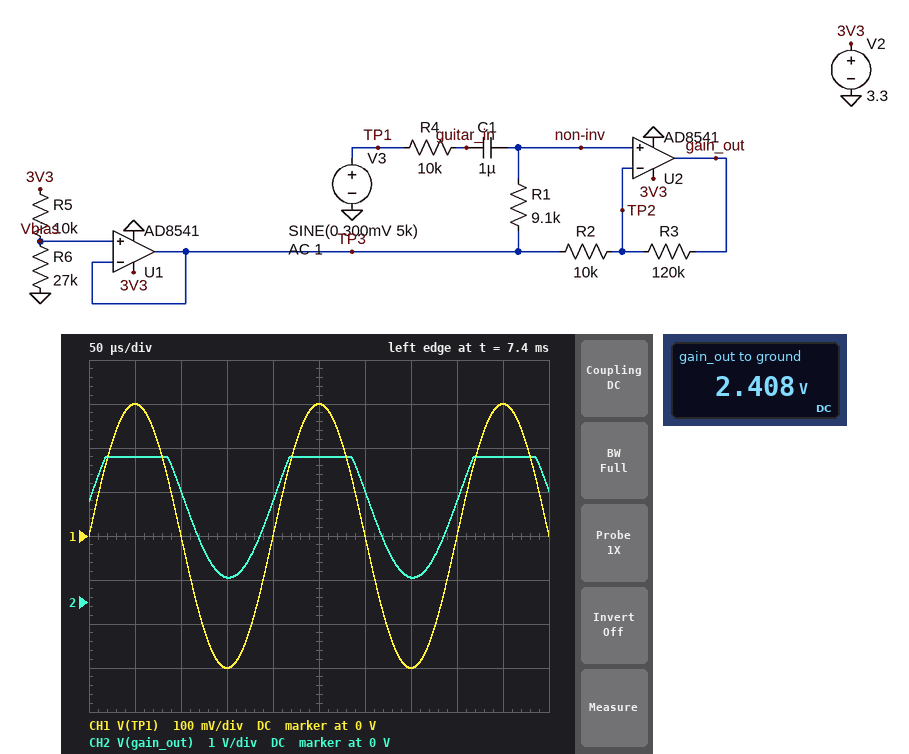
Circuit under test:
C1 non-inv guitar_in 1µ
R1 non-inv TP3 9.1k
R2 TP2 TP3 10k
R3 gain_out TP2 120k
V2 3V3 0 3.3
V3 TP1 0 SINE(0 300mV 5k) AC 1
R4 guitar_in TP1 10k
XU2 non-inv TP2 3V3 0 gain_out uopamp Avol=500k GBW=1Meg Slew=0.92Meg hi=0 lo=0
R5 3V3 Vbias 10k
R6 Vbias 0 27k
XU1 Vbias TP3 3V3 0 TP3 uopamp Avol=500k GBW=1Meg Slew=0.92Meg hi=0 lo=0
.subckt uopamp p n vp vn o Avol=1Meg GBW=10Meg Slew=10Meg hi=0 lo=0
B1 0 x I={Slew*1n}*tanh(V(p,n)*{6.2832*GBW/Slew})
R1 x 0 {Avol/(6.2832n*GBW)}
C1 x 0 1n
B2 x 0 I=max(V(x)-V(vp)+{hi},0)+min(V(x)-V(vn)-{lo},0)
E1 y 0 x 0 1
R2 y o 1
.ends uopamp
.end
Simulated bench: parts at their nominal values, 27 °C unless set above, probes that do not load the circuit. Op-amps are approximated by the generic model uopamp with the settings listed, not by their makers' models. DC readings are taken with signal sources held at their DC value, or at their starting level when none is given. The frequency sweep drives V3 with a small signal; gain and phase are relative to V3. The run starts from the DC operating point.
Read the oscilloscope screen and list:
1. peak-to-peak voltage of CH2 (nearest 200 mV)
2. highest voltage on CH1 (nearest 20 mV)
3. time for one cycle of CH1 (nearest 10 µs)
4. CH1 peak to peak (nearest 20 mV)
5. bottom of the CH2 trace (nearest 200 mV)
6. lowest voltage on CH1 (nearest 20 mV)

2.8 V
300 mV
200 µs
600 mV
600 mV
-300 mV
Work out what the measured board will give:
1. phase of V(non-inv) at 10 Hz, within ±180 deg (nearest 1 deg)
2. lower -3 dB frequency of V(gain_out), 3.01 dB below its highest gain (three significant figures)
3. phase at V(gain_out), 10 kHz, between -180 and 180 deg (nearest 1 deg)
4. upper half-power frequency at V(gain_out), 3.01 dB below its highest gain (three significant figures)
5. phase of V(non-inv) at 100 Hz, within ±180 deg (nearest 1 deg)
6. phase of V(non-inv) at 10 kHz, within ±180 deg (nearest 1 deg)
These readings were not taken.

40 deg
8.33 Hz
-7 deg
76.9 kHz
5 deg
0 deg
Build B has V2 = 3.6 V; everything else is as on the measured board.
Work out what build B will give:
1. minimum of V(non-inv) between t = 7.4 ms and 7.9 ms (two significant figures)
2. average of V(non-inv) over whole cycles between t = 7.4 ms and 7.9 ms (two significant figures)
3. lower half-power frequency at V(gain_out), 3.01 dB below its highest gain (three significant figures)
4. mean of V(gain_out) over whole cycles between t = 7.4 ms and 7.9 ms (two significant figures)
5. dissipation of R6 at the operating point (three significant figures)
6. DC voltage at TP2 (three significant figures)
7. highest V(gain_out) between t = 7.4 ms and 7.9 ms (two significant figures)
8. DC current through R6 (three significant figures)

2.5 V
2.6 V
8.33 Hz
2.4 V
256 µW
2.63 V
3.6 V
97.3 µA
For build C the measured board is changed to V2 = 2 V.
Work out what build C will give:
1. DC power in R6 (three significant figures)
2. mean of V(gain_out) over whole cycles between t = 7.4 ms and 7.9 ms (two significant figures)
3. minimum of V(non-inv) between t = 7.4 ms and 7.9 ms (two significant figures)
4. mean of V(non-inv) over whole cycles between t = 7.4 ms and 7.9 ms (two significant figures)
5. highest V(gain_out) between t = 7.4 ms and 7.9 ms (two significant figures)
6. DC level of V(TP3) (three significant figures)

78.9 µW
1.2 V
1.3 V
1.5 V
2.0 V
1.46 V
